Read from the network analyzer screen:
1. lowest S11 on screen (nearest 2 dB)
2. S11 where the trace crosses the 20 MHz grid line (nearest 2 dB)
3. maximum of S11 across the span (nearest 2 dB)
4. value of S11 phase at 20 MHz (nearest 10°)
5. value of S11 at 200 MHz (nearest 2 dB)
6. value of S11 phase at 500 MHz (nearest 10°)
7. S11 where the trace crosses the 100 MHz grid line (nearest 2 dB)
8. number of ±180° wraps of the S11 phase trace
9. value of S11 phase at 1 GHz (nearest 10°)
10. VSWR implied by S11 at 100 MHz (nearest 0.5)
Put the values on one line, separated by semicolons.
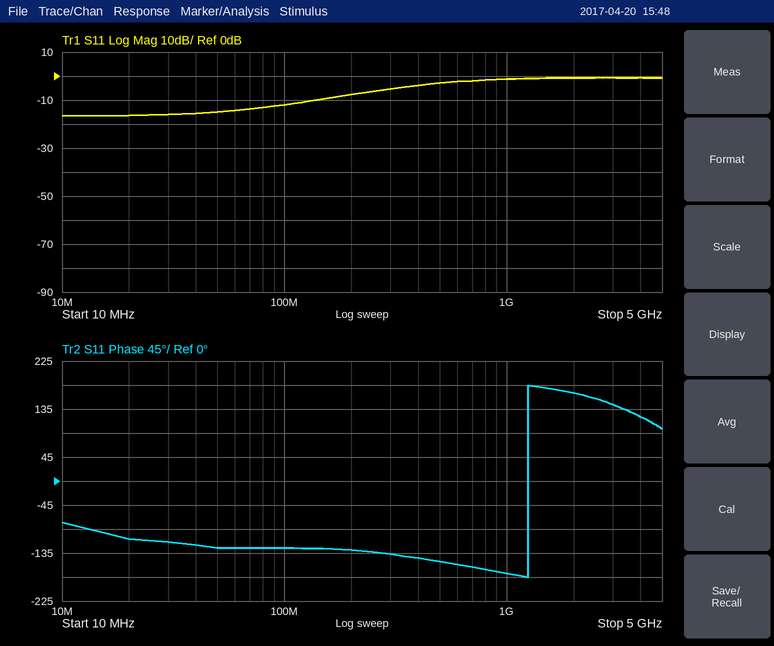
-16 dB; -16 dB; 0 dB; -110°; -8 dB; -150°; -12 dB; 1; -170°; 1.5
